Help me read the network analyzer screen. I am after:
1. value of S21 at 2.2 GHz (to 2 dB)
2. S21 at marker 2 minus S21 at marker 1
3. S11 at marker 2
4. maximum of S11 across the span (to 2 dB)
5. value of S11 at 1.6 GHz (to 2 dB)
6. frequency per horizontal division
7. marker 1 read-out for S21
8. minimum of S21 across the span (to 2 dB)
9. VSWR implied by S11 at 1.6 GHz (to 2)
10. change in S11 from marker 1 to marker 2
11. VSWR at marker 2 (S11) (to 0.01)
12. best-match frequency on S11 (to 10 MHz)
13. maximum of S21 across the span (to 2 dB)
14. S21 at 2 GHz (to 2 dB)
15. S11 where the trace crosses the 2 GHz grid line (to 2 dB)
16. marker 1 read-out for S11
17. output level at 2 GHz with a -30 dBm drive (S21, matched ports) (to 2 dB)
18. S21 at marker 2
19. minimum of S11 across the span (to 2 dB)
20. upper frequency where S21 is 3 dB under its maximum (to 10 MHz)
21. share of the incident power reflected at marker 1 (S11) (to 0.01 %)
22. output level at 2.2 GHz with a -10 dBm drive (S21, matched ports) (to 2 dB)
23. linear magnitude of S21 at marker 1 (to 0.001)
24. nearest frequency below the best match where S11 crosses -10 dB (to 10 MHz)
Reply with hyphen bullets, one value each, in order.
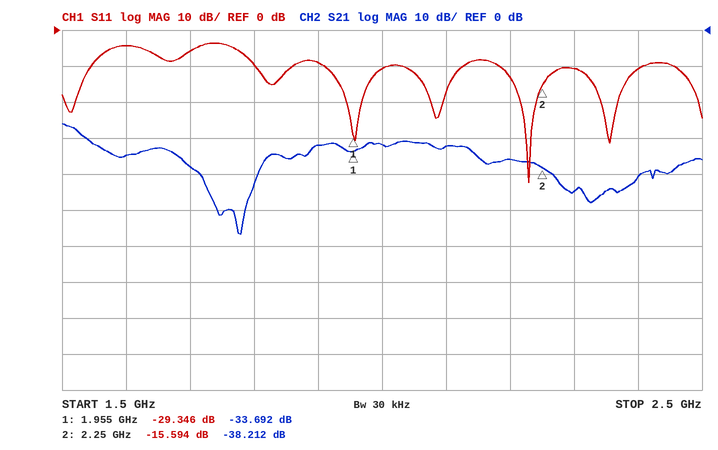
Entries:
- -36 dB
- -4.520 dB
- -15.594 dB
- -4 dB
- -4 dB
- 100 MHz
- -33.692 dB
- -56 dB
- 4
- 13.752 dB
- 1.40
- 2.23 GHz
- -26 dB
- -32 dB
- -10 dB
- -29.346 dB
- -62 dBm
- -38.212 dB
- -42 dB
- 1.53 GHz
- 0.12 %
- -46 dBm
- 0.021
- 2.18 GHz
